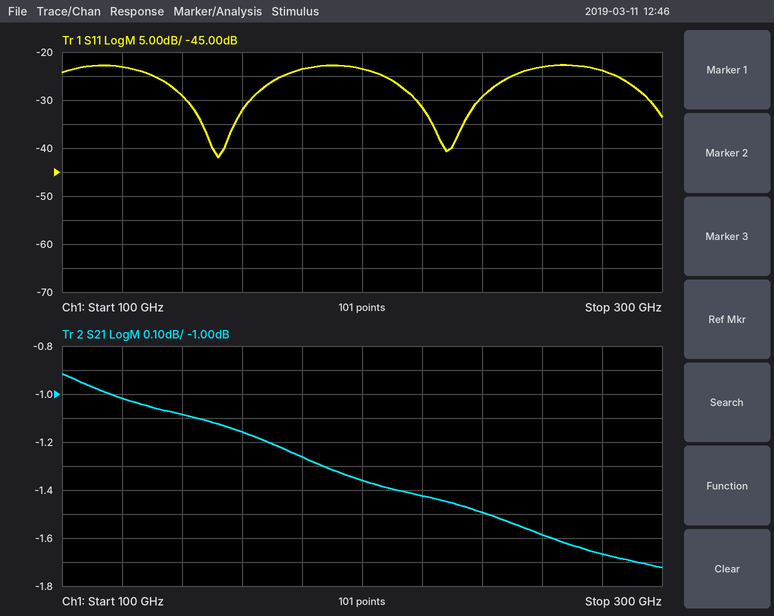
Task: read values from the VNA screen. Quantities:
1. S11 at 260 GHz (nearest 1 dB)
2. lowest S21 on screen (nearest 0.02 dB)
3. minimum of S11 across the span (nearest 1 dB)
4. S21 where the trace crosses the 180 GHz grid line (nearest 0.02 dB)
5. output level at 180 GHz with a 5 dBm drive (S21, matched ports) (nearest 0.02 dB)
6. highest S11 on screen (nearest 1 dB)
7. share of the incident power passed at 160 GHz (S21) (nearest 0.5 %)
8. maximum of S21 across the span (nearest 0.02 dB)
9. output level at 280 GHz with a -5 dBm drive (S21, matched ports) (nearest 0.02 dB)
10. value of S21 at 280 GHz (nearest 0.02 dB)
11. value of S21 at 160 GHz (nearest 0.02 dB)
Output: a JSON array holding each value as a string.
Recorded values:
["-23 dB", "-1.72 dB", "-42 dB", "-1.26 dB", "3.74 dBm", "-23 dB", "76.5 %", "-0.92 dB", "-6.66 dBm", "-1.66 dB", "-1.16 dB"]
